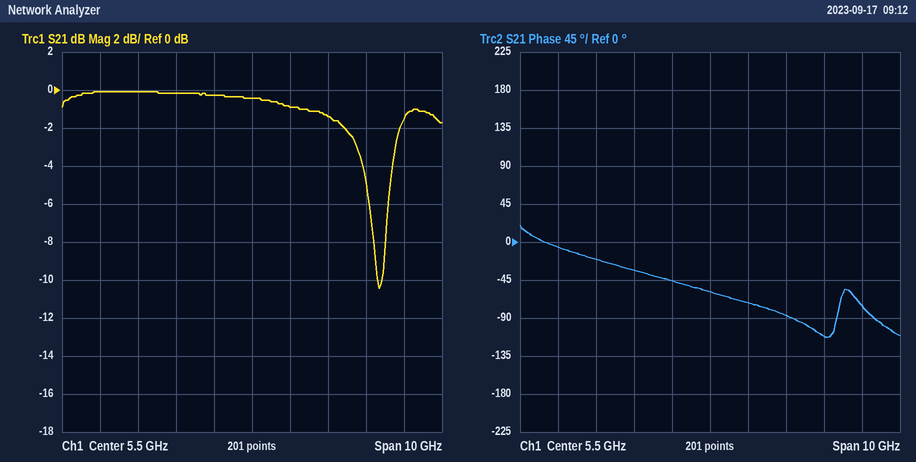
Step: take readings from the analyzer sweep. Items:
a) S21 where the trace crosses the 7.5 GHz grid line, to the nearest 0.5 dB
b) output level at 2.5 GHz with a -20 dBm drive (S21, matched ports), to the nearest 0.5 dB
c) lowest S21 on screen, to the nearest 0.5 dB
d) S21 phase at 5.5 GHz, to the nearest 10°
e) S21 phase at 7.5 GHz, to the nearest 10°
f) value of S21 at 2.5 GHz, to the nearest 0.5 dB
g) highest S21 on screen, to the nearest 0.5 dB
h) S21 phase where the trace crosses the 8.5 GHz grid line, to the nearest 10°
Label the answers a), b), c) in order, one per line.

a) -1.5 dB
b) -20.0 dBm
c) -10.5 dB
d) -60°
e) -90°
f) 0.0 dB
g) 0.0 dB
h) -110°
